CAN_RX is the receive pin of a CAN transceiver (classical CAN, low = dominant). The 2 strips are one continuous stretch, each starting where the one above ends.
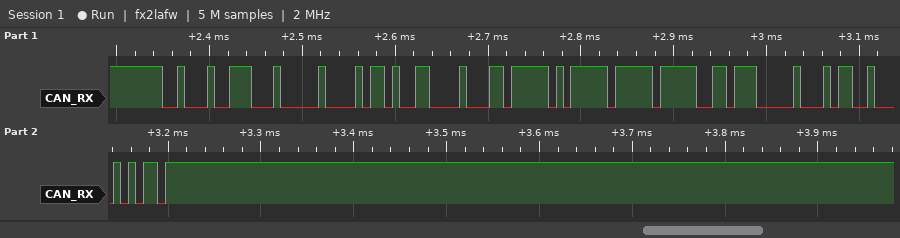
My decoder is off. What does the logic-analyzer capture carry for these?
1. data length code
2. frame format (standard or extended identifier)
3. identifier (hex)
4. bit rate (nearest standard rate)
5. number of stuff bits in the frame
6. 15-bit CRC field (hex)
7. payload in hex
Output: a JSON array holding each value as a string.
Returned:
["8", "standard", "0x227", "125 kbit/s", "6", "0x5915", "02 D3 08 DF BF FF B7 00"]
